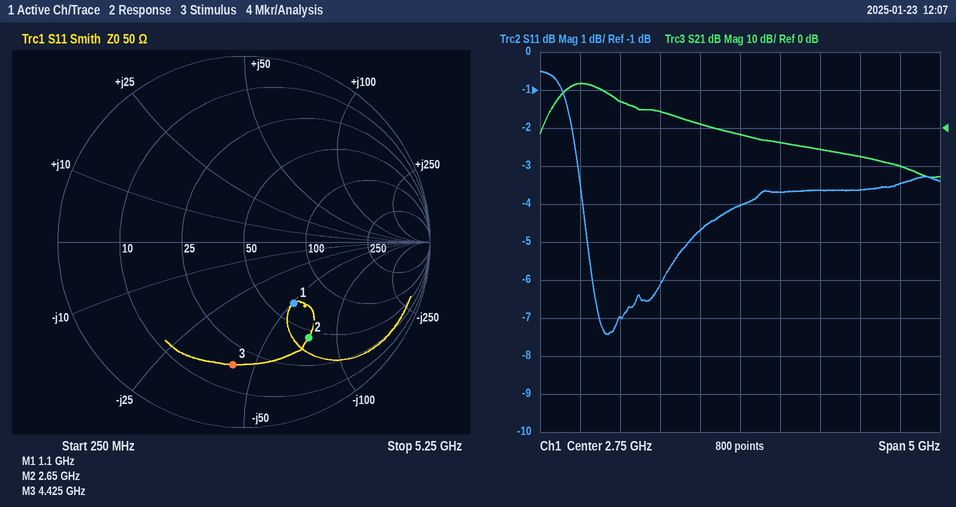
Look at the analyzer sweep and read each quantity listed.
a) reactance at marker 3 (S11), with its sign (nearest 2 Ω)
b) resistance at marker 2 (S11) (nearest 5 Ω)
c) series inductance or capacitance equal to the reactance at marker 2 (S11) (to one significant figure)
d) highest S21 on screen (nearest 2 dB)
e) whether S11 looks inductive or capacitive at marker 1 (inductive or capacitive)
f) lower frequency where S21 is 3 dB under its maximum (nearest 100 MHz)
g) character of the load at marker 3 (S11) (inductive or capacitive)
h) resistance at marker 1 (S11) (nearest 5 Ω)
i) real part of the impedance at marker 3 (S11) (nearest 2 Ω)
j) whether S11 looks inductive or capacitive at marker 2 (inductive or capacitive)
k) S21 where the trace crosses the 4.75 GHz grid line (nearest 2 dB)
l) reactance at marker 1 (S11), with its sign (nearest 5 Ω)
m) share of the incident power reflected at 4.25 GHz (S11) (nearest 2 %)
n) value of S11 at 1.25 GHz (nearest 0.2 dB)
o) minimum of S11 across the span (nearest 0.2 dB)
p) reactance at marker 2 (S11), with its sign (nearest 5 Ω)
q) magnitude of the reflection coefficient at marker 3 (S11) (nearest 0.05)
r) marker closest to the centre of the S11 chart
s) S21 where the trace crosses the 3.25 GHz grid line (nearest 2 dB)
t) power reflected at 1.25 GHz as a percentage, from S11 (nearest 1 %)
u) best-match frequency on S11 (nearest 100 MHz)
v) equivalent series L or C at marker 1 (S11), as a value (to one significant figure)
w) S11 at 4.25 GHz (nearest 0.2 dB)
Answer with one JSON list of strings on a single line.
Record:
["-42 Ω", "45 Ω", "800 fF", "12 dB", "capacitive", "500 MHz", "capacitive", "65 Ω", "18 Ω", "capacitive", "-10 dB", "-50 Ω", "44 %", "-7.0 dB", "-7.4 dB", "-75 Ω", "0.65", "marker 1", "-4 dB", "20 %", "1.1 GHz", "3 pF", "-3.6 dB"]
